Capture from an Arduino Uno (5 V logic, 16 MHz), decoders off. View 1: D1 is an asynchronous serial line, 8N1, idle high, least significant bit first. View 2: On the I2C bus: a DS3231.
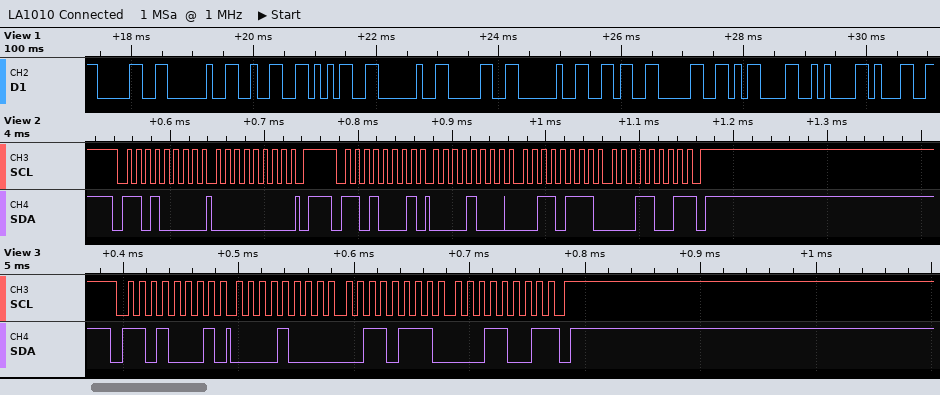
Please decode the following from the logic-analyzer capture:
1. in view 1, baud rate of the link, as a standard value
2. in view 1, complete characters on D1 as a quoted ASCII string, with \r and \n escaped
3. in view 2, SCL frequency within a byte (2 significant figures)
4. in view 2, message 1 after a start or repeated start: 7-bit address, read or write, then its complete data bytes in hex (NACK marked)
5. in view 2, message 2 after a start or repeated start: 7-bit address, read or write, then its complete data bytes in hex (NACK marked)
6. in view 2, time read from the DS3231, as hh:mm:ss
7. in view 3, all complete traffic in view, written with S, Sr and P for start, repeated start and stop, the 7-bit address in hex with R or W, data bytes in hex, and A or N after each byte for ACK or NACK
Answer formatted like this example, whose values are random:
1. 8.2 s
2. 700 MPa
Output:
1. 9600 baud
2. "0 25 0 60\r\n1"
3. 100 kHz
4. 0x68 write: 00
5. 0x68 read: 08 37 19 NACK
6. 19:37:08
7. S 68R A 08 A 37 A 19 N P
